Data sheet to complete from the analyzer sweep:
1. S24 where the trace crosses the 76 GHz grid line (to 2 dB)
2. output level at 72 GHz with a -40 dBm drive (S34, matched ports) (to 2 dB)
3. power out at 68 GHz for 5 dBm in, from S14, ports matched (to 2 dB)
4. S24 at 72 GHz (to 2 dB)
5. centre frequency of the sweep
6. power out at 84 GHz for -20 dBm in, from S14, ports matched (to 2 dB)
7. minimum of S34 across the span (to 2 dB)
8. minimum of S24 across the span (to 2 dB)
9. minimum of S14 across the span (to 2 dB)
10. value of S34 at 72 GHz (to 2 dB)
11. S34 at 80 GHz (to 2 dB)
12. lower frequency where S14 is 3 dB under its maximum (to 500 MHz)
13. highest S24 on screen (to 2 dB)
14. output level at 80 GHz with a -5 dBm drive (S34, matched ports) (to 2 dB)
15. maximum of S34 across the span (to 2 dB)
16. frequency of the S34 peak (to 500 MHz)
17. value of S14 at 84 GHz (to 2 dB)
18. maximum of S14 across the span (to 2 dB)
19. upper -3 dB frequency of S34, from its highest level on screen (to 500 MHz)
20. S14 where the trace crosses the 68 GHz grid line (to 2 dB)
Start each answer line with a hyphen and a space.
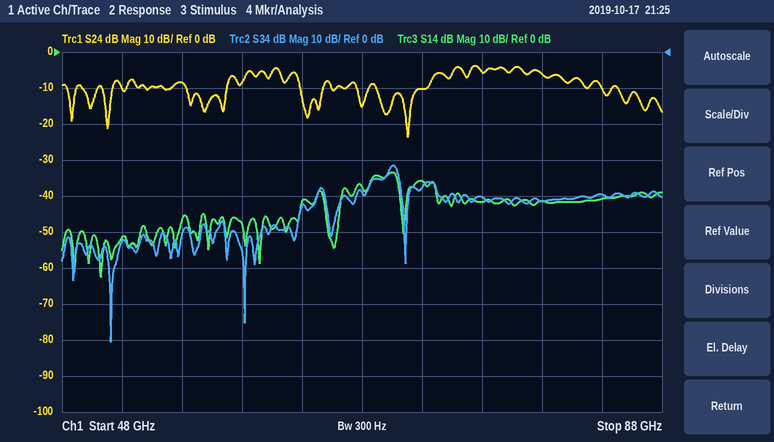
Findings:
- -6 dB
- -78 dBm
- -32 dBm
- -10 dB
- 68 GHz
- -60 dBm
- -80 dB
- -24 dB
- -62 dB
- -38 dB
- -42 dB
- 68.5 GHz
- -4 dB
- -46 dBm
- -32 dB
- 70.0 GHz
- -40 dB
- -34 dB
- 70.5 GHz
- -38 dB
